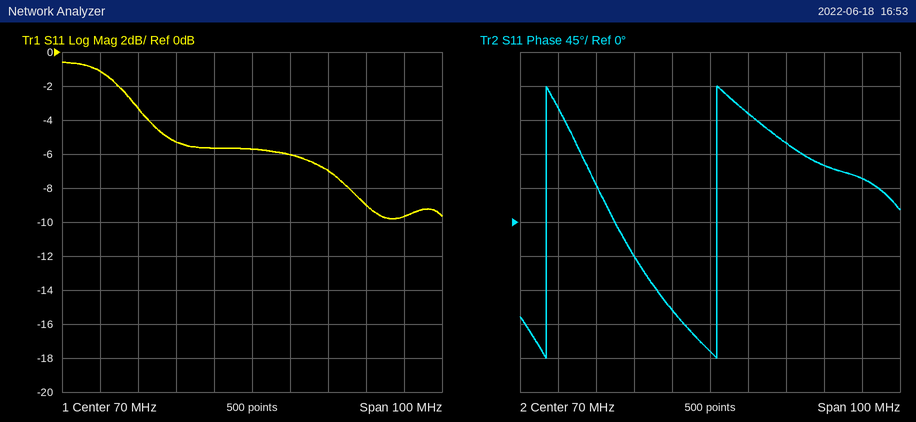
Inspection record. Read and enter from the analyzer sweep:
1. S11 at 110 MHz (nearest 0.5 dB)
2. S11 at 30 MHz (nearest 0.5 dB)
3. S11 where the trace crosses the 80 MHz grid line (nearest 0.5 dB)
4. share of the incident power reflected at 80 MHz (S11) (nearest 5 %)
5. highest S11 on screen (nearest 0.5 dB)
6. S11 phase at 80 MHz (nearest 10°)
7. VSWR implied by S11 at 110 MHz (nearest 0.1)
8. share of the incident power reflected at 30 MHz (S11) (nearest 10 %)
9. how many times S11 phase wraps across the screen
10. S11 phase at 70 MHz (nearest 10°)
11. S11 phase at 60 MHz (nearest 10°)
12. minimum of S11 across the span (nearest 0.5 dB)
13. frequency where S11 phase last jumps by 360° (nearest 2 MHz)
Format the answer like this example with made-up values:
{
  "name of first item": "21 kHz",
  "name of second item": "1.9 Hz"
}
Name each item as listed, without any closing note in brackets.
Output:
{
  "S11 at 110 MHz": "-9.5 dB",
  "S11 at 30 MHz": "-1.0 dB",
  "S11 where the trace crosses the 80 MHz grid line": "-6.0 dB",
  "share of the incident power reflected at 80 MHz (S11)": "25 %",
  "highest S11 on screen": "-0.5 dB",
  "S11 phase at 80 MHz": "140°",
  "VSWR implied by S11 at 110 MHz": "2.0",
  "share of the incident power reflected at 30 MHz (S11)": "80 %",
  "how many times S11 phase wraps across the screen": "2",
  "S11 phase at 70 MHz": "-170°",
  "S11 phase at 60 MHz": "-120°",
  "minimum of S11 across the span": "-10.0 dB",
  "frequency where S11 phase last jumps by 360°": "72 MHz"
}
